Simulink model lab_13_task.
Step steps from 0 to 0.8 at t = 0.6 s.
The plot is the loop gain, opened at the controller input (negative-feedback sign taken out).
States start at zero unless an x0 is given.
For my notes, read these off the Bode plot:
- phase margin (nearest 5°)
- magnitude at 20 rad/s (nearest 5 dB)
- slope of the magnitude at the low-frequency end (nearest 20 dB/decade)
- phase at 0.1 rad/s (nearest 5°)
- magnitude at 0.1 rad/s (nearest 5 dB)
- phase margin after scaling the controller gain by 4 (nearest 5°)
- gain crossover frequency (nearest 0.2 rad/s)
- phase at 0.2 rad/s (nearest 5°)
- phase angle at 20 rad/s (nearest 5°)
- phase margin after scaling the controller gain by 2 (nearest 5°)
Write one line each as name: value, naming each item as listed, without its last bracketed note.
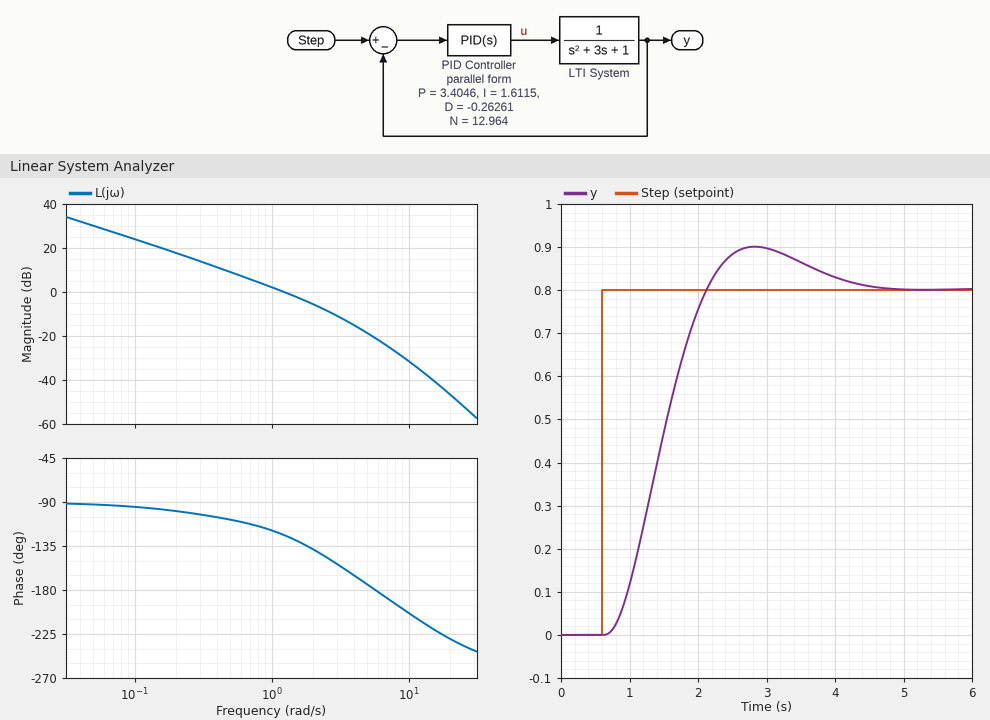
phase margin: 55°
magnitude at 20 rad/s: -45 dB
slope of the magnitude at the low-frequency end: -20 dB/decade
phase at 0.1 rad/s: -95°
magnitude at 0.1 rad/s: 25 dB
phase margin after scaling the controller gain by 4: 25°
gain crossover frequency: 1.2 rad/s
phase at 0.2 rad/s: -100°
phase angle at 20 rad/s: -230°
phase margin after scaling the controller gain by 2: 40°
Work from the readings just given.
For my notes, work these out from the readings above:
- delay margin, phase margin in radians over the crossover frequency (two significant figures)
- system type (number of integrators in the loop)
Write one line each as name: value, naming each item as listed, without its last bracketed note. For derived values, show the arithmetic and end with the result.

delay margin, phase margin in radians over the crossover frequency: 55 × π / 180 / 1.2 = 0.80 s
system type: 1
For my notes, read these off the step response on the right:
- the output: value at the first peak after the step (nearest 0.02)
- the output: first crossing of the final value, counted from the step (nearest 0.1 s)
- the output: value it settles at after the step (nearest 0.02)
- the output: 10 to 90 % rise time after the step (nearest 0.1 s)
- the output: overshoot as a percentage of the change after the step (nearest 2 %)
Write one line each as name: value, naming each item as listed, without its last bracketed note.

the output: value at the first peak after the step: 0.90
the output: first crossing of the final value, counted from the step: 1.5 s
the output: value it settles at after the step: 0.80
the output: 10 to 90 % rise time after the step: 1.0 s
the output: overshoot as a percentage of the change after the step: 12 %
